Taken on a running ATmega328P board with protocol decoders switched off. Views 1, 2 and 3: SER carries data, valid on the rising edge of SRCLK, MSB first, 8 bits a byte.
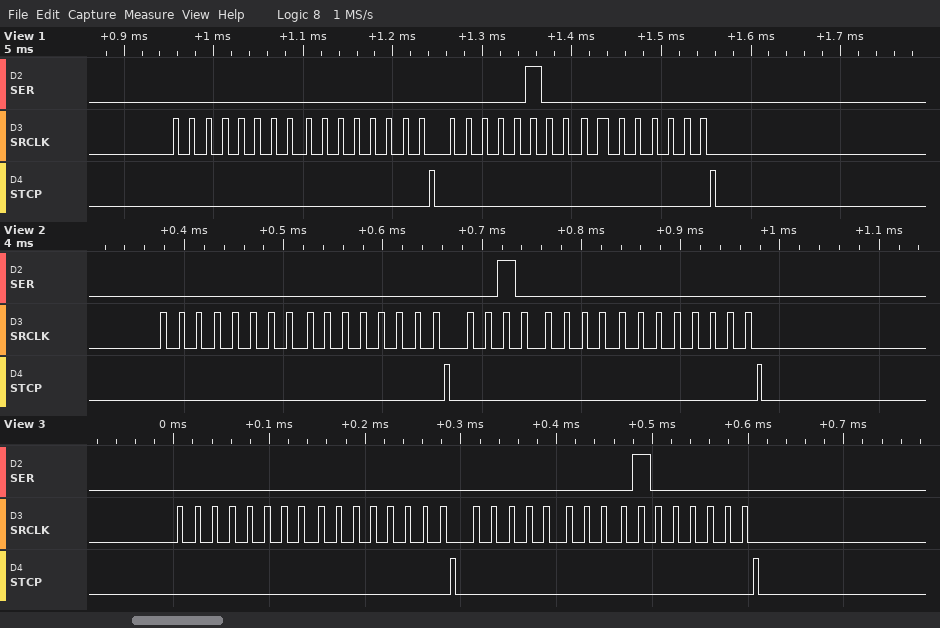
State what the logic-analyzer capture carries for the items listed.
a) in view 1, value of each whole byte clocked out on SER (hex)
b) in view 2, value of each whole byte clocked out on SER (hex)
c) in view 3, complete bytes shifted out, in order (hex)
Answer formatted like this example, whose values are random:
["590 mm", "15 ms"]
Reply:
["0x00 0x00 0x04 0x00", "00 00 20 00", "0x00 0x00 0x00 0x40"]
